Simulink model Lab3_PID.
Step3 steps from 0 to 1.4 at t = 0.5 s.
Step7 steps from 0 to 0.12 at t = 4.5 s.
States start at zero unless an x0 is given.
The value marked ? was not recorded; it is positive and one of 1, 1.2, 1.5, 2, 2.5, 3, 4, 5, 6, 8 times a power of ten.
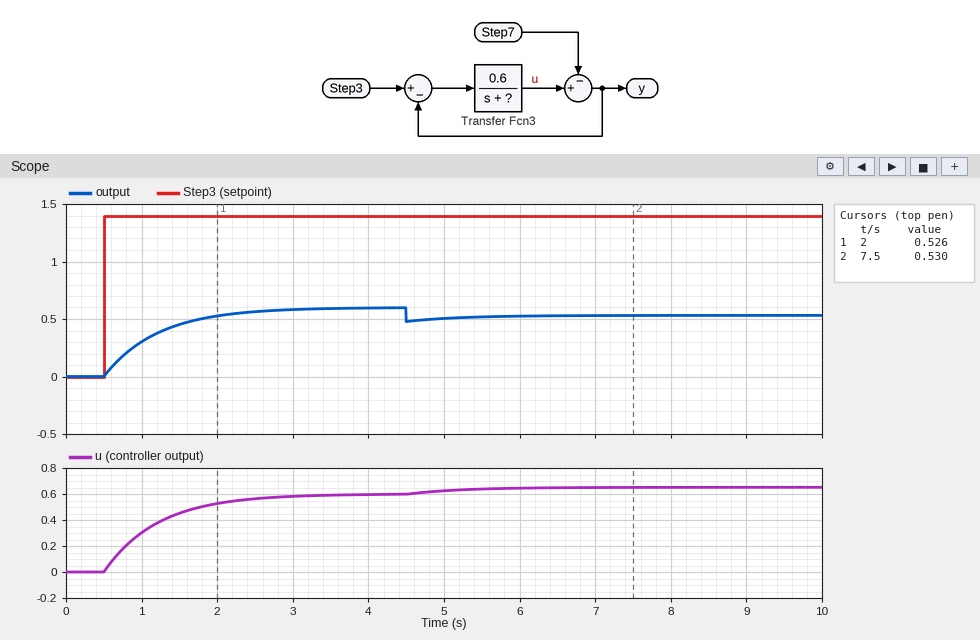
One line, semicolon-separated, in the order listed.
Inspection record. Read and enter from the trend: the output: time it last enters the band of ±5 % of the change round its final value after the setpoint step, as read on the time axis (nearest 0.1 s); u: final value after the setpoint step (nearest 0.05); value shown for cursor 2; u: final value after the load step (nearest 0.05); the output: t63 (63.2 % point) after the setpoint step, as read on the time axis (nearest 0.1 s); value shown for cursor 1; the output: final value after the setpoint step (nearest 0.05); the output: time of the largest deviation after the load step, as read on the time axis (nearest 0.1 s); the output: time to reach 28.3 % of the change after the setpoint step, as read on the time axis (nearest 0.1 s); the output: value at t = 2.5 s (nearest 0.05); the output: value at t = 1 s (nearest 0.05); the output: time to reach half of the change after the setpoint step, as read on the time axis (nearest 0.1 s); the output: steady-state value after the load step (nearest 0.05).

2.6 s; 0.60; 0.530; 0.65; 1.2 s; 0.526; 0.60; 4.5 s; 0.7 s; 0.55; 0.30; 1.0 s; 0.55
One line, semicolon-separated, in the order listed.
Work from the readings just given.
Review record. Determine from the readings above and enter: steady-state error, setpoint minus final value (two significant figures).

0.80
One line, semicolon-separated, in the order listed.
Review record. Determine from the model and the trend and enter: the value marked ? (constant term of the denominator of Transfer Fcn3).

0.8
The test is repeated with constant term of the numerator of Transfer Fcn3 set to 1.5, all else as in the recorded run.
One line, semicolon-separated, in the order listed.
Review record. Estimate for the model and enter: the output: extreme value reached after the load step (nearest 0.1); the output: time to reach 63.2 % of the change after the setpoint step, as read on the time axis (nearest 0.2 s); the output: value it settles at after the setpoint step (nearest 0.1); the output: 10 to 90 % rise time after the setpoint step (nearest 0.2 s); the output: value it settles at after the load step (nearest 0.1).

0.8; 1.0 s; 0.9; 1.0 s; 0.9
